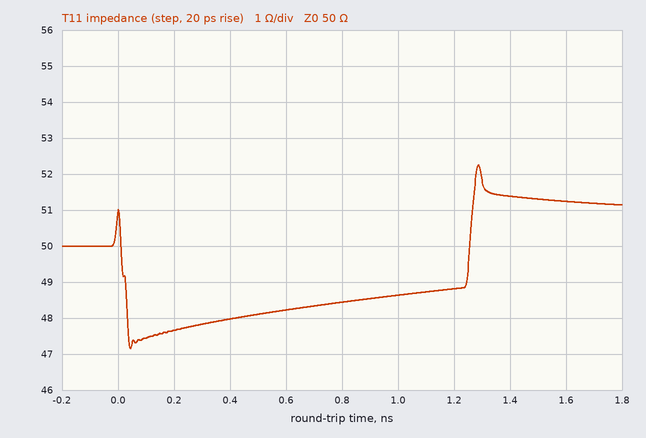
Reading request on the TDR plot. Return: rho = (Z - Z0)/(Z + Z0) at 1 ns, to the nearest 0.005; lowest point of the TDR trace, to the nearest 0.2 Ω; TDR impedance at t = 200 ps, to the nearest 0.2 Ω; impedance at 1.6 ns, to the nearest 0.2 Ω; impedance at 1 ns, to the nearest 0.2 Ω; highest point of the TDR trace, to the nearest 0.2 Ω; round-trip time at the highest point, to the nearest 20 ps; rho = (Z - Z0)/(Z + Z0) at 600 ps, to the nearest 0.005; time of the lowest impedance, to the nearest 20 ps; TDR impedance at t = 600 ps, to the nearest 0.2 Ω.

-0.015
47.2 Ω
47.6 Ω
51.2 Ω
48.6 Ω
52.2 Ω
1.28 ns
-0.020
40 ps
48.2 Ω
